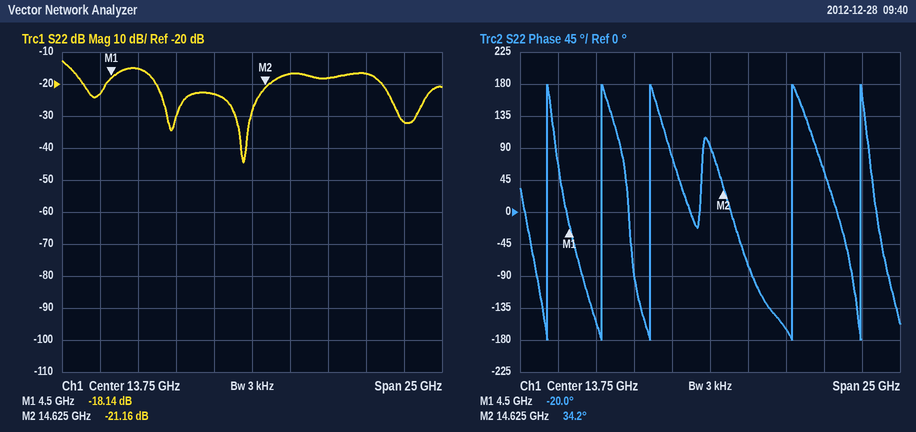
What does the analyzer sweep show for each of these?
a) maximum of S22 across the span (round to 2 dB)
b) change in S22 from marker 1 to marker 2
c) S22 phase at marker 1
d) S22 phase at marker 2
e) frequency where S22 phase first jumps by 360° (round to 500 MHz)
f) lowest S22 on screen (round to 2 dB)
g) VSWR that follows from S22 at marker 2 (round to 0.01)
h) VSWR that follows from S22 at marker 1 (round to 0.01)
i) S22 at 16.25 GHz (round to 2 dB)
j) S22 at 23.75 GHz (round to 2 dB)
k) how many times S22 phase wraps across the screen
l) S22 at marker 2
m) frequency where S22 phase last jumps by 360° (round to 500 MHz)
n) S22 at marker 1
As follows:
-12 dB
-3.02 dB
-20.0°
34.2°
3.0 GHz
-44 dB
1.19
1.28
-16 dB
-32 dB
5
-21.16 dB
23.5 GHz
-18.14 dB
